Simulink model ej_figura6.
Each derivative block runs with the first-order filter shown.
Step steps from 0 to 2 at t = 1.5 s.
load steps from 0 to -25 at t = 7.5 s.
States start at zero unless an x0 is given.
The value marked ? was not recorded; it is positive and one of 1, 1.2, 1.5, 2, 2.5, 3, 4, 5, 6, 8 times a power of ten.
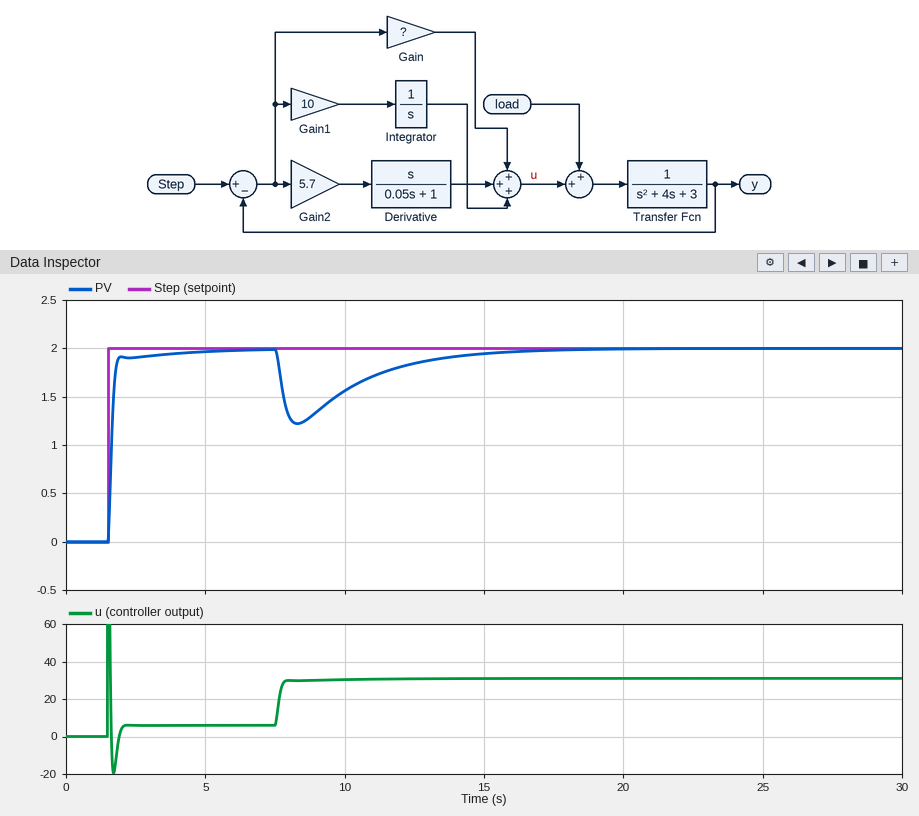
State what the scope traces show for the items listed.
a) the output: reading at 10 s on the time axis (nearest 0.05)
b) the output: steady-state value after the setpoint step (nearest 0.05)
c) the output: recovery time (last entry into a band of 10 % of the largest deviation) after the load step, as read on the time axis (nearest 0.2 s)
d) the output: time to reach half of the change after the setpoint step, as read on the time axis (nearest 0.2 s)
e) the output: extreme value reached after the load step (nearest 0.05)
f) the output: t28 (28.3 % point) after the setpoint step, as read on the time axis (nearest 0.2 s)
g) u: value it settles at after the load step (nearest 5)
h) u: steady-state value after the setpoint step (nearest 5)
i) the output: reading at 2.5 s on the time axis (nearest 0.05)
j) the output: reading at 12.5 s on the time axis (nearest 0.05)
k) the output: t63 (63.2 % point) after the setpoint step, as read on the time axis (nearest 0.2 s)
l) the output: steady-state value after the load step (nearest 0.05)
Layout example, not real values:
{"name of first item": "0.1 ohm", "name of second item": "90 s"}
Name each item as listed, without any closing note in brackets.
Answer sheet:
{"the output: reading at 10 s on the time axis": "1.55", "the output: steady-state value after the setpoint step": "2.00", "the output: recovery time (last entry into a band of 10 % of the largest deviation) after the load step, as read on the time axis": "14.2 s", "the output: time to reach half of the change after the setpoint step, as read on the time axis": "1.6 s", "the output: extreme value reached after the load step": "1.20", "the output: t28 (28.3 % point) after the setpoint step, as read on the time axis": "1.6 s", "u: value it settles at after the load step": "30", "u: steady-state value after the setpoint step": "5", "the output: reading at 2.5 s on the time axis": "1.90", "the output: reading at 12.5 s on the time axis": "1.85", "the output: t63 (63.2 % point) after the setpoint step, as read on the time axis": "1.6 s", "the output: steady-state value after the load step": "2.00"}
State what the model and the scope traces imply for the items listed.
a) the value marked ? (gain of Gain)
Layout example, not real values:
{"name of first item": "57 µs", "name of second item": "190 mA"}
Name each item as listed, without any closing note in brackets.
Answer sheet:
{"the value marked ?": "25"}
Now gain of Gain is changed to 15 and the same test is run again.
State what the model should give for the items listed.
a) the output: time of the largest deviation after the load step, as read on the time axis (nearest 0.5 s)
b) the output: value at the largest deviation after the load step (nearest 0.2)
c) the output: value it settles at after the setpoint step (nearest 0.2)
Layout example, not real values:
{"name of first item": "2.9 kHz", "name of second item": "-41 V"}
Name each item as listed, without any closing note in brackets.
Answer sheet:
{"the output: time of the largest deviation after the load step, as read on the time axis": "8.5 s", "the output: value at the largest deviation after the load step": "1.0", "the output: value it settles at after the setpoint step": "2.0"}
